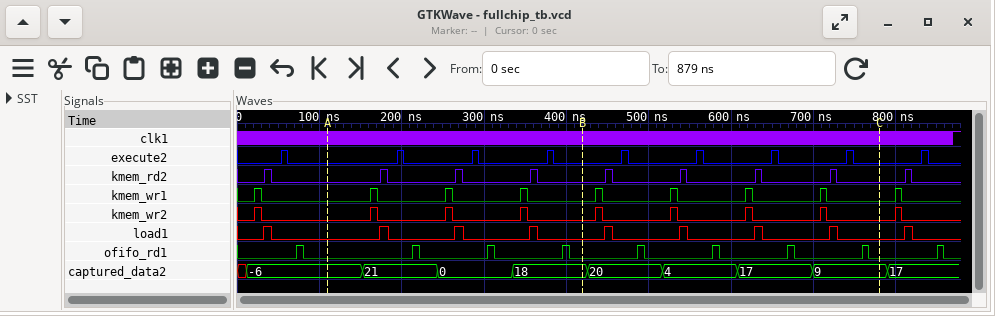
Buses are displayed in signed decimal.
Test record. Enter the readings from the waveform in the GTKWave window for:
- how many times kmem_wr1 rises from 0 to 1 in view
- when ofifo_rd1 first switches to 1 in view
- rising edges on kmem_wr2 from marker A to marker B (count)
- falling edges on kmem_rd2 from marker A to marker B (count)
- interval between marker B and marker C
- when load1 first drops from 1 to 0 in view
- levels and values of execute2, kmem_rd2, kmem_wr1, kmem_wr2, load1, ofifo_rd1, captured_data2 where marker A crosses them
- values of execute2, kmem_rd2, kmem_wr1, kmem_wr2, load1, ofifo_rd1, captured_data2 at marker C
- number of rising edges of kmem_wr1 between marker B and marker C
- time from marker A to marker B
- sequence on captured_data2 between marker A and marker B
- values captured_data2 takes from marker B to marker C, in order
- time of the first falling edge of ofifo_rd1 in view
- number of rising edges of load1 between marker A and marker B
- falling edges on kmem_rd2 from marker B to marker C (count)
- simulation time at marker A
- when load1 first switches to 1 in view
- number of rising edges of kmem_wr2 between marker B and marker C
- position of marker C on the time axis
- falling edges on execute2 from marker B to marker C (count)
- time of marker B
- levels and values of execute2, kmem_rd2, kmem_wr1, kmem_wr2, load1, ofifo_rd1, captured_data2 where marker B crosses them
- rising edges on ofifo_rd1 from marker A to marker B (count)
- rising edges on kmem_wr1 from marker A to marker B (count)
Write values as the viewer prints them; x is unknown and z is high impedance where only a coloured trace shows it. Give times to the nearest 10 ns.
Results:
9
70 ns
3
3
360 ns
40 ns
execute2=0, kmem_rd2=0, kmem_wr1=0, kmem_wr2=0, load1=0, ofifo_rd1=0, captured_data2=-6
execute2=0, kmem_rd2=0, kmem_wr1=0, kmem_wr2=0, load1=0, ofifo_rd1=0, captured_data2=9
4
310 ns
-6, 21, 0, 18
18, 20, 4, 17, 9
80 ns
3
4
110 ns
30 ns
4
780 ns
4
420 ns
execute2=0, kmem_rd2=0, kmem_wr1=0, kmem_wr2=0, load1=0, ofifo_rd1=0, captured_data2=18
3
3
